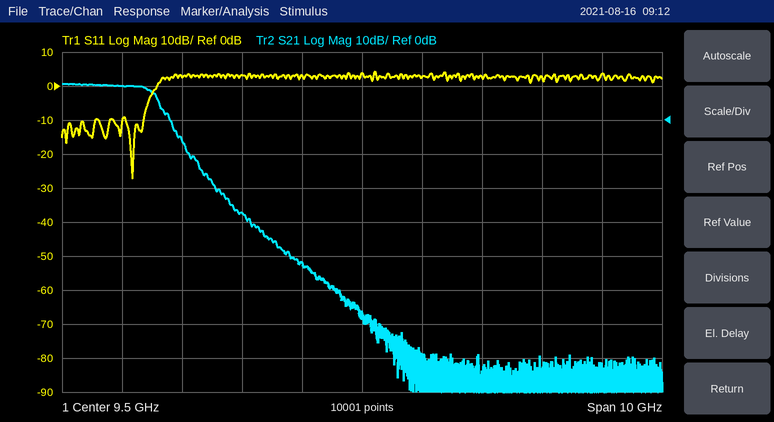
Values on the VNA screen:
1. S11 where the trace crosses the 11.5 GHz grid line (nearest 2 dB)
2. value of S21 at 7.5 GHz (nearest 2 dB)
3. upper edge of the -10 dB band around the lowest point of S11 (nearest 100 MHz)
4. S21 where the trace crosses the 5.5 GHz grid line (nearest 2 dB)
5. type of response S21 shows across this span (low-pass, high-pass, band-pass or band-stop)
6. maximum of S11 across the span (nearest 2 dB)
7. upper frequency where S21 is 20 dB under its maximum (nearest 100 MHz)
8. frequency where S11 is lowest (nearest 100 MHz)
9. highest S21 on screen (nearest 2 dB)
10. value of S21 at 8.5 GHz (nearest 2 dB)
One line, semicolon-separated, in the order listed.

2 dB; -28 dB; 5.9 GHz; 10 dB; low-pass; 4 dB; 6.6 GHz; 5.7 GHz; 10 dB; -42 dB
